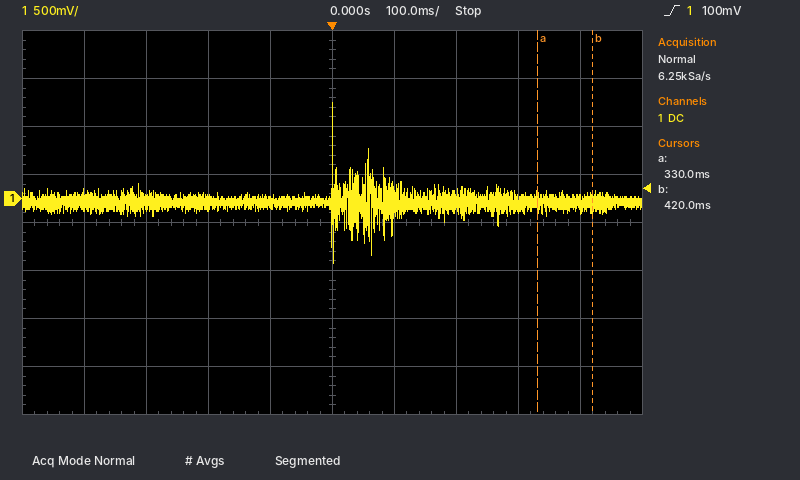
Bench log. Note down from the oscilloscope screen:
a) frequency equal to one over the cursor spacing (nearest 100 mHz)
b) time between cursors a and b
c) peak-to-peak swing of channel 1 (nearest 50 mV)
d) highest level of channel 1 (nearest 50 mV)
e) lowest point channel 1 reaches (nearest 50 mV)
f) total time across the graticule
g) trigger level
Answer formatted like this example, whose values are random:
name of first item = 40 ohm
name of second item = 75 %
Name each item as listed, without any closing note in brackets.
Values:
frequency equal to one over the cursor spacing = 11.1 Hz
time between cursors a and b = 90 ms
peak-to-peak swing of channel 1 = 1.65 V
highest level of channel 1 = 1.00 V
lowest point channel 1 reaches = -650 mV
total time across the graticule = 1 s
trigger level = 100 mV
